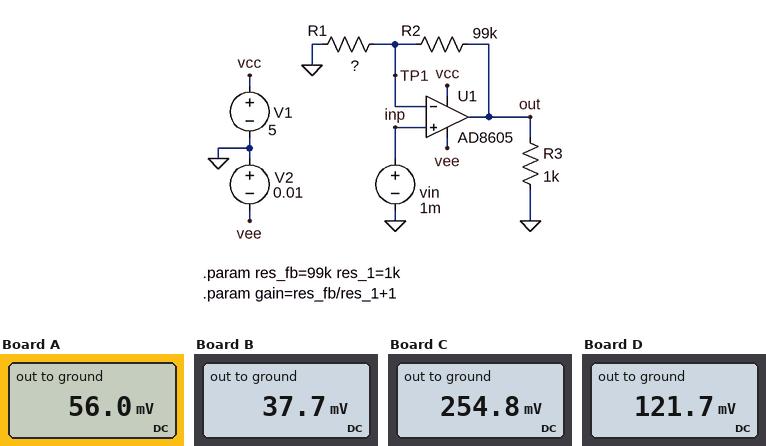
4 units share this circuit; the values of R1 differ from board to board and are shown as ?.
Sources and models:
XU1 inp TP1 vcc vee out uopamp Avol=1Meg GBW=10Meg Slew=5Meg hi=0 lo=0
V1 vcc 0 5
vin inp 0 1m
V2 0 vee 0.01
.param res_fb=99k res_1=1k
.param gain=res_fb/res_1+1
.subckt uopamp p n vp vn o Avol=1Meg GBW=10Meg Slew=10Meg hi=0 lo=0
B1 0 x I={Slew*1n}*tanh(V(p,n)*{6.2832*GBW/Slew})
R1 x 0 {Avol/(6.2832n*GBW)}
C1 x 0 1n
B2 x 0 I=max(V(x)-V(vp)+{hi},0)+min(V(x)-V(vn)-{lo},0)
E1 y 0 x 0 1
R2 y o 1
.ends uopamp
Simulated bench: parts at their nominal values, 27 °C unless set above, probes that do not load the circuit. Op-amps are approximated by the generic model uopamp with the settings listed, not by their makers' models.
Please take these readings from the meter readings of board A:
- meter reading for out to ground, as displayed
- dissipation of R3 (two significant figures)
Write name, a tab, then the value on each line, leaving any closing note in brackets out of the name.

meter reading for out to ground, as displayed	56.0 mV
dissipation of R3	3.1 µW
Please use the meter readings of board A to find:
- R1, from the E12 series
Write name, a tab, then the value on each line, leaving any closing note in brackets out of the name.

R1, from the E12 series	1.8 kΩ
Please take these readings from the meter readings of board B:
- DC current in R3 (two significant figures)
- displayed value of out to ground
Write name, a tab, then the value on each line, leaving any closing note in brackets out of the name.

DC current in R3	38 µA
displayed value of out to ground	37.7 mV
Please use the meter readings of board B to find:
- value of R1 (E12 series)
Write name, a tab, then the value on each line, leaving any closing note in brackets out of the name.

value of R1	2.7 kΩ
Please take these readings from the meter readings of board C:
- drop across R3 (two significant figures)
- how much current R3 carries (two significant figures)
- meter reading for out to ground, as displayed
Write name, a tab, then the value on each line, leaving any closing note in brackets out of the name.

drop across R3	250 mV
how much current R3 carries	250 µA
meter reading for out to ground, as displayed	254.8 mV
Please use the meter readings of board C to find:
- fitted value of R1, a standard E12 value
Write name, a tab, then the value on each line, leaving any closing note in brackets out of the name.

fitted value of R1, a standard E12 value	390 Ω
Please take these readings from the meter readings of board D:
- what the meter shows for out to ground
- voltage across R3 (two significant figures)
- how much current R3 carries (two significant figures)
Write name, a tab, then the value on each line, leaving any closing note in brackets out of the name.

what the meter shows for out to ground	121.7 mV
voltage across R3	120 mV
how much current R3 carries	120 µA
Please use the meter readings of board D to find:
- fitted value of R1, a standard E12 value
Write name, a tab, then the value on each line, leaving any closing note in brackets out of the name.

fitted value of R1, a standard E12 value	820 Ω
